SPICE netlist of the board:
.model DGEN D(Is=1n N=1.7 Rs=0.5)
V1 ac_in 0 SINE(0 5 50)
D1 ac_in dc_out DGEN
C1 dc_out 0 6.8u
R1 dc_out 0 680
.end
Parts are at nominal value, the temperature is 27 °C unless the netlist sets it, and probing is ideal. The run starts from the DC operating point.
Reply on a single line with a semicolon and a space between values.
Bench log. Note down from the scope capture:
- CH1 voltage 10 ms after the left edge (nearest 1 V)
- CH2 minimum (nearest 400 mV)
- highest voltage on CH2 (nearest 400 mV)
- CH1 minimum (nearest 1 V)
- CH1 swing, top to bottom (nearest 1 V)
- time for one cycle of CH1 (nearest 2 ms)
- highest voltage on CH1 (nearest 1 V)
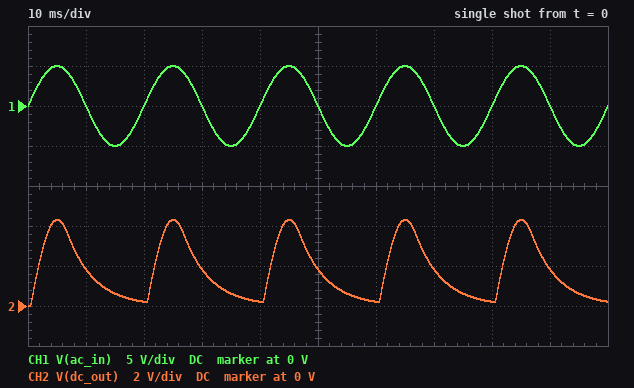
0 V; 0 V; 4.4 V; -5 V; 10 V; 20 ms; 5 V
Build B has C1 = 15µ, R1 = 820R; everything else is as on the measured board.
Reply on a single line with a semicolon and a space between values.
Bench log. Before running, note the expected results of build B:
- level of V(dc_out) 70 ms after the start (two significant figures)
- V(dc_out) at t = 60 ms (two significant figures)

3.0 V; 1.3 V
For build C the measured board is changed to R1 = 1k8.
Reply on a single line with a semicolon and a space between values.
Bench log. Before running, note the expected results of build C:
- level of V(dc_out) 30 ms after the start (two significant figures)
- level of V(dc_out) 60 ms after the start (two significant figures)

3.0 V; 1.3 V
